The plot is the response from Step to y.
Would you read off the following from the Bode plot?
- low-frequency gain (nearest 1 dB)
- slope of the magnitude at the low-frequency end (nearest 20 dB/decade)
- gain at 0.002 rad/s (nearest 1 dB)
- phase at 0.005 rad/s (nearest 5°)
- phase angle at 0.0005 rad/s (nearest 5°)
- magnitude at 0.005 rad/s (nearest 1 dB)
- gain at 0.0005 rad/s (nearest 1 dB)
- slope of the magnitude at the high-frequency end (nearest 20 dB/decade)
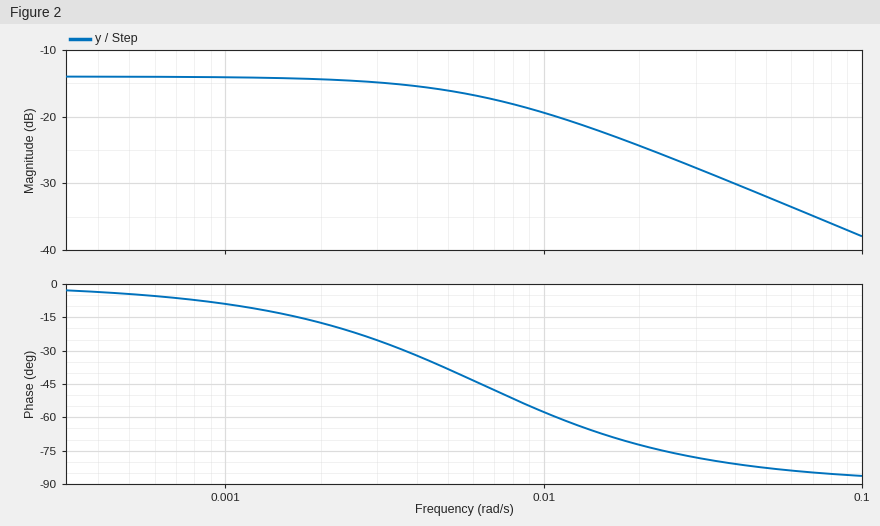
-14 dB
0 dB/decade
-14 dB
-40°
-5°
-16 dB
-14 dB
-20 dB/decade
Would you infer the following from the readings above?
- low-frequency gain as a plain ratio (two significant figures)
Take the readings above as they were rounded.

0.20
